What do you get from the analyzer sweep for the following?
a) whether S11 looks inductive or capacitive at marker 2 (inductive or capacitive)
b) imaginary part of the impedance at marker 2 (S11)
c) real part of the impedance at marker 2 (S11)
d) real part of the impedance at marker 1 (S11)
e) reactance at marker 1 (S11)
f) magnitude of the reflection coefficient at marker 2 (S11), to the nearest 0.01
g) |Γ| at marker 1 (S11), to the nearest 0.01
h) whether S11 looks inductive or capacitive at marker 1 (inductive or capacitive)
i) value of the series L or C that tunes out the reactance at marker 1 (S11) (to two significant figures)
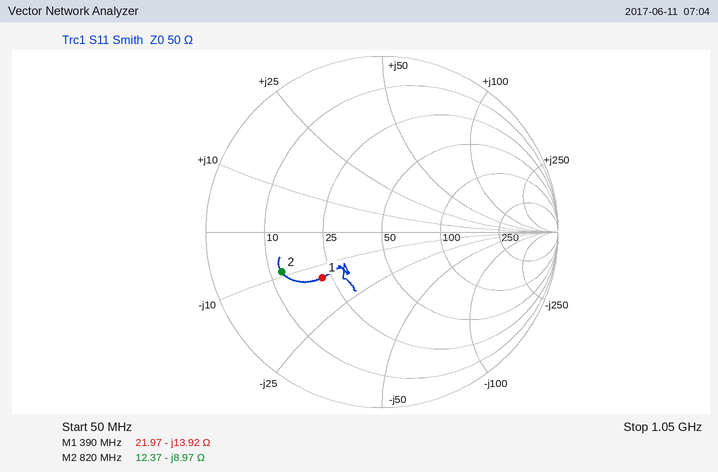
capacitive
-8.97 Ω
12.37 Ω
21.97 Ω
-13.92 Ω
0.61
0.43
capacitive
5.7 nH
